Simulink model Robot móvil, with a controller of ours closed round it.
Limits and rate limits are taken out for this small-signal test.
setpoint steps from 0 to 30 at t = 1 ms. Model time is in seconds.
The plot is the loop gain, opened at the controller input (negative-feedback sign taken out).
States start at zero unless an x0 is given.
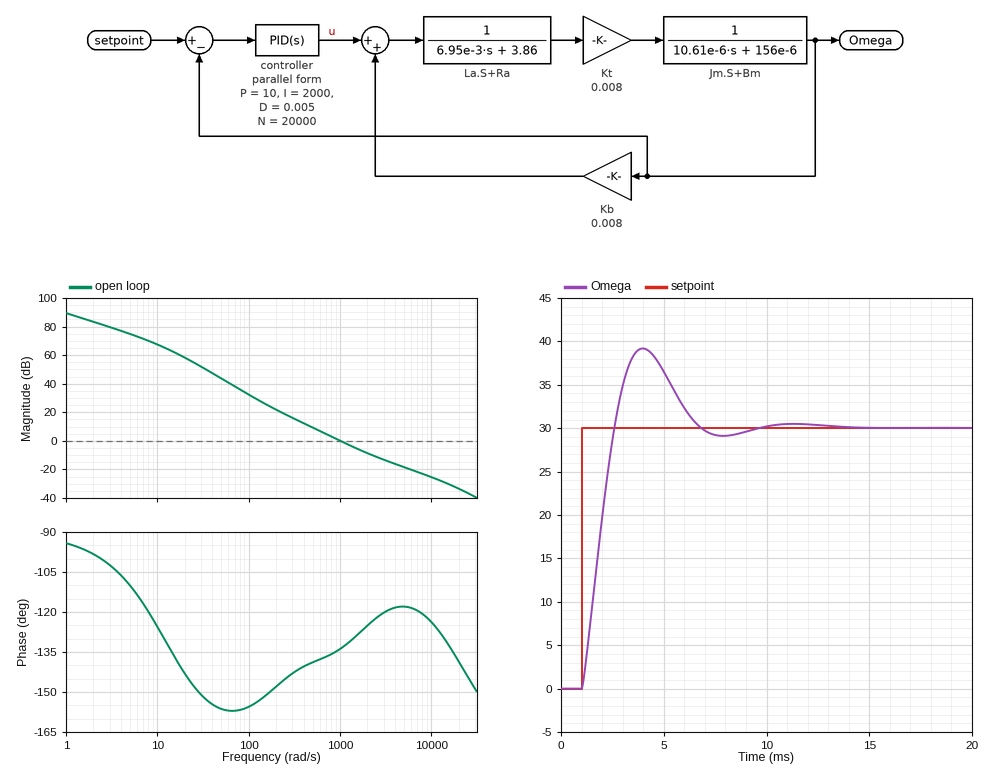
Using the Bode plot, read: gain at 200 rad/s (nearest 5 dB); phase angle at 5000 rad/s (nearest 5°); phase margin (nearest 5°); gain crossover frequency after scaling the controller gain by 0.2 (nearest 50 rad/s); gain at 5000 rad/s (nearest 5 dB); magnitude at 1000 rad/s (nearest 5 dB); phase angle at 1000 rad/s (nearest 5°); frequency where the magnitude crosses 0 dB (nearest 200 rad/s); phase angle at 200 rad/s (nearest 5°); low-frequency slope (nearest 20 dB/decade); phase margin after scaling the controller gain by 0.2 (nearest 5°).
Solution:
20 dB
-120°
45°
350 rad/s
-20 dB
0 dB
-135°
1000 rad/s
-150°
-20 dB/decade
40°
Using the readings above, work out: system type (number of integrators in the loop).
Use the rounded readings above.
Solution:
1
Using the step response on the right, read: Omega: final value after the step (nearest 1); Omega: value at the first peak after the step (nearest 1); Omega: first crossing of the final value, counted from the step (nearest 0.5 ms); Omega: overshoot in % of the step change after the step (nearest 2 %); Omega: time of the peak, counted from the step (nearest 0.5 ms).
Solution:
30
39
1.5 ms
30 %
3.0 ms
